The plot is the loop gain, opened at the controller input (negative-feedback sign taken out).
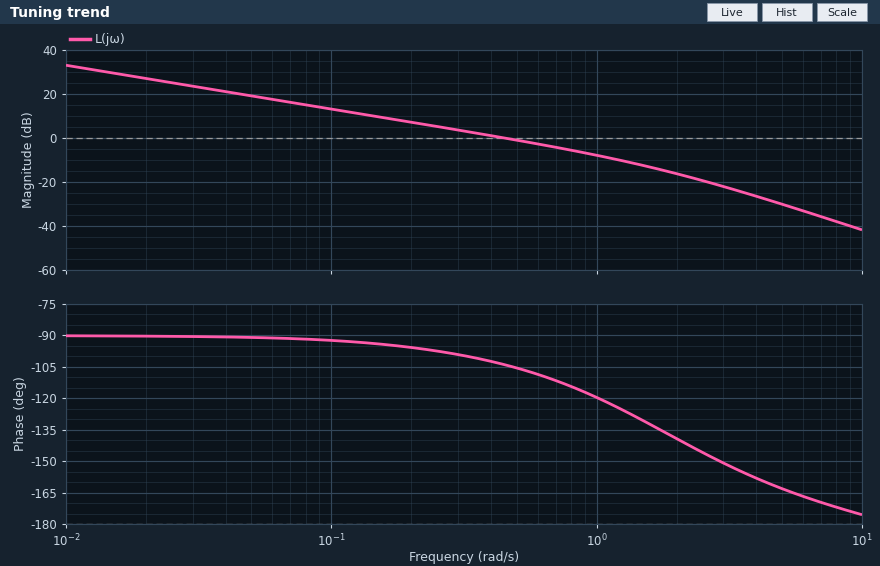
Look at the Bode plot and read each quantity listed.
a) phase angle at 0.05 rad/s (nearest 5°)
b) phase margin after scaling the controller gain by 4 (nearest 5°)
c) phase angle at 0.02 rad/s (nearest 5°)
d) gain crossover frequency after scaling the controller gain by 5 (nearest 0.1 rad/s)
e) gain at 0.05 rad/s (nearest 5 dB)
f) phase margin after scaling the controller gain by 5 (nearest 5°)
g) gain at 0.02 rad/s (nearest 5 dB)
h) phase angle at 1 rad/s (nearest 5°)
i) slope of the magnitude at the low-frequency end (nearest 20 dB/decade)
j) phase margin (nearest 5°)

-90°
50°
-90°
1.7 rad/s
20 dB
45°
25 dB
-120°
-20 dB/decade
75°
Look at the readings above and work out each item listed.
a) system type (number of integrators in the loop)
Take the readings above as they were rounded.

1
